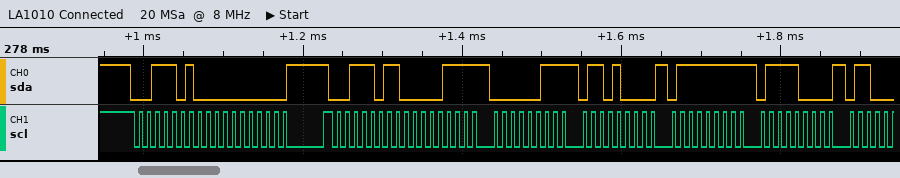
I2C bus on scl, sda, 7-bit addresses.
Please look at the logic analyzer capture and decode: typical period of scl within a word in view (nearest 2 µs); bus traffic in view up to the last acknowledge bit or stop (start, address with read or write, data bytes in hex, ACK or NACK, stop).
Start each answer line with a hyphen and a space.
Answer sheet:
- 10 µs
- start, address 1D write ACK, 00 ACK, repeated start, address 1D read ACK, 0F ACK, 07 ACK, D0 ACK, FF ACK, F0 ACK
